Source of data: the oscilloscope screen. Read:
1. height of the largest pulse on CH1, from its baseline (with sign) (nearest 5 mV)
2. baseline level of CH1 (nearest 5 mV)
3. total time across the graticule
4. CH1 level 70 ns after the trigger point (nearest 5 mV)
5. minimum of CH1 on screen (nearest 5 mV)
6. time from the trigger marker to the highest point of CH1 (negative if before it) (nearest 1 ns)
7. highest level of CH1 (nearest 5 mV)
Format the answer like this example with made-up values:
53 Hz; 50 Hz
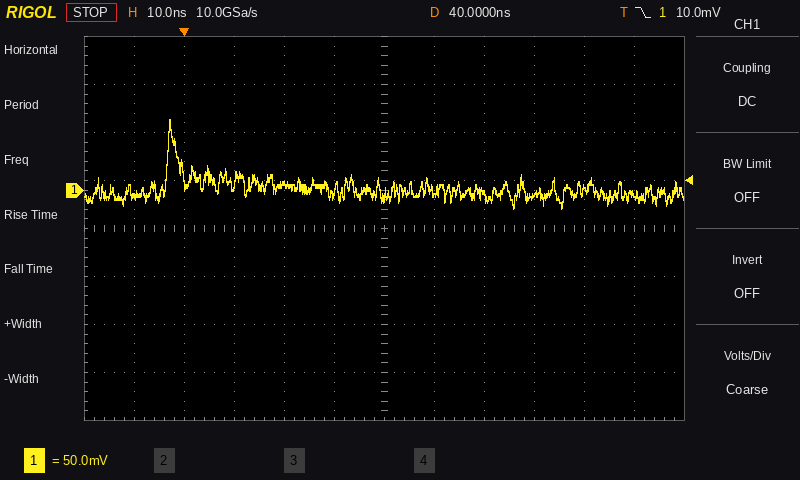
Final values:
+75 mV; 0 mV; 120 ns; -5 mV; -20 mV; -3 ns; 75 mV
